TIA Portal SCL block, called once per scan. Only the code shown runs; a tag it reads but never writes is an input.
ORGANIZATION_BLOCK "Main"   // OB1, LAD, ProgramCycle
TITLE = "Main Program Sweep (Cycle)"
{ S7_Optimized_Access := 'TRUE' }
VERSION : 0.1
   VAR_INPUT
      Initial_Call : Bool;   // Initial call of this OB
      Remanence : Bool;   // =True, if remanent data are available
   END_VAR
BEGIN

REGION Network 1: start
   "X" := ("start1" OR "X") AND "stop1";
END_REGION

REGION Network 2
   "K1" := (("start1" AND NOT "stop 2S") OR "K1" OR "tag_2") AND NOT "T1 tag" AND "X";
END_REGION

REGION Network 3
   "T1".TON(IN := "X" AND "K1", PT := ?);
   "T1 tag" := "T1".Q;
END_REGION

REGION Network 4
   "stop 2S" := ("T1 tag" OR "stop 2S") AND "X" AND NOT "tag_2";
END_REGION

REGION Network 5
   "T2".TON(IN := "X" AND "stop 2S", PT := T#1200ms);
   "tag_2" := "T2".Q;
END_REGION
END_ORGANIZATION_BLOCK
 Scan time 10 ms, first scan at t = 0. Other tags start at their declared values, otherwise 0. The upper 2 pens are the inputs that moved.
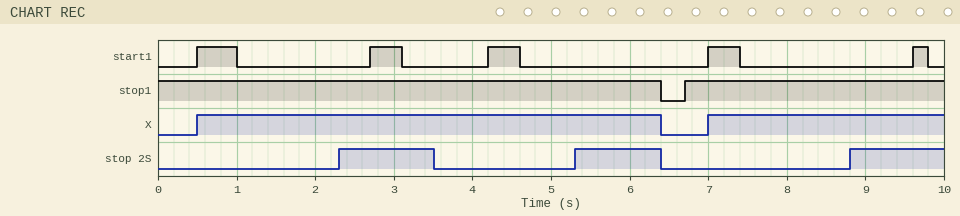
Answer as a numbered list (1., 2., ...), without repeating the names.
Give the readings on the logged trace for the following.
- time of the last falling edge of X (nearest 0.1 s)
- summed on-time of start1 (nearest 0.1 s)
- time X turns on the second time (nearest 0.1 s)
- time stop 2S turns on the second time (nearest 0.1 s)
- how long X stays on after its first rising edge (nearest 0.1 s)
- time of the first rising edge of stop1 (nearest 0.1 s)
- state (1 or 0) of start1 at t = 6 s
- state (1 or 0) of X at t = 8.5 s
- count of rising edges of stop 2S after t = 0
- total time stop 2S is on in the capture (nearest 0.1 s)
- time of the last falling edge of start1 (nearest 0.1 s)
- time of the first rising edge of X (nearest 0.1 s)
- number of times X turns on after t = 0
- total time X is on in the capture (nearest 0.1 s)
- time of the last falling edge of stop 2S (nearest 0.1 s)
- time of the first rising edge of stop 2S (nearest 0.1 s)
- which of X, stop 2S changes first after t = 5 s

1. 6.4 s
2. 1.9 s
3. 7.0 s
4. 5.3 s
5. 5.9 s
6. 6.7 s
7. 0
8. 1
9. 3
10. 3.5 s
11. 9.8 s
12. 0.5 s
13. 2
14. 8.9 s
15. 6.4 s
16. 2.3 s
17. stop 2S
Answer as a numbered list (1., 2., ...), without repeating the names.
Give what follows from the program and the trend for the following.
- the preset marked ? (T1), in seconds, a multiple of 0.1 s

1. 1.8 s
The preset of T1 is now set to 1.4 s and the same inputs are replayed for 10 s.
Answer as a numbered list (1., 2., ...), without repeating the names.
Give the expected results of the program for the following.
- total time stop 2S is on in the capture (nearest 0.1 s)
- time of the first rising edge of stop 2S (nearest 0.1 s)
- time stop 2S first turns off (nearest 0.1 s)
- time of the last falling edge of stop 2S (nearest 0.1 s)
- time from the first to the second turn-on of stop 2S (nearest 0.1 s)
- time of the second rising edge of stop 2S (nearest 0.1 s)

1. 3.6 s
2. 1.9 s
3. 3.1 s
4. 9.6 s
5. 2.6 s
6. 4.5 s
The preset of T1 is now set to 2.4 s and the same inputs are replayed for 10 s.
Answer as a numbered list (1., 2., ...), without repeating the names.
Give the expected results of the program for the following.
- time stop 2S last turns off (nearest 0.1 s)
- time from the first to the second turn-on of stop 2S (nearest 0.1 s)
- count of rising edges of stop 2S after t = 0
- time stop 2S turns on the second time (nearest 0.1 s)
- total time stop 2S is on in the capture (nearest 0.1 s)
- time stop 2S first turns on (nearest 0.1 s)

1. 4.1 s
2. 6.5 s
3. 2
4. 9.4 s
5. 1.8 s
6. 2.9 s
